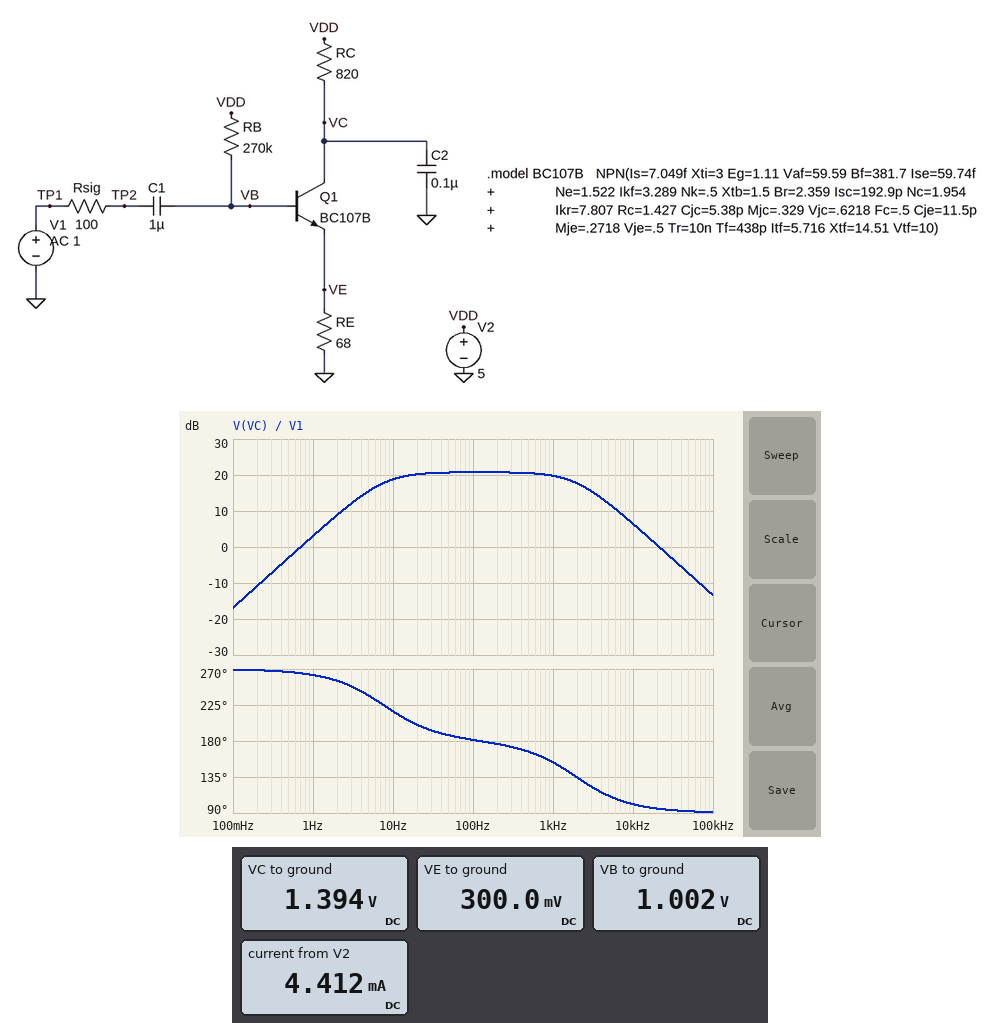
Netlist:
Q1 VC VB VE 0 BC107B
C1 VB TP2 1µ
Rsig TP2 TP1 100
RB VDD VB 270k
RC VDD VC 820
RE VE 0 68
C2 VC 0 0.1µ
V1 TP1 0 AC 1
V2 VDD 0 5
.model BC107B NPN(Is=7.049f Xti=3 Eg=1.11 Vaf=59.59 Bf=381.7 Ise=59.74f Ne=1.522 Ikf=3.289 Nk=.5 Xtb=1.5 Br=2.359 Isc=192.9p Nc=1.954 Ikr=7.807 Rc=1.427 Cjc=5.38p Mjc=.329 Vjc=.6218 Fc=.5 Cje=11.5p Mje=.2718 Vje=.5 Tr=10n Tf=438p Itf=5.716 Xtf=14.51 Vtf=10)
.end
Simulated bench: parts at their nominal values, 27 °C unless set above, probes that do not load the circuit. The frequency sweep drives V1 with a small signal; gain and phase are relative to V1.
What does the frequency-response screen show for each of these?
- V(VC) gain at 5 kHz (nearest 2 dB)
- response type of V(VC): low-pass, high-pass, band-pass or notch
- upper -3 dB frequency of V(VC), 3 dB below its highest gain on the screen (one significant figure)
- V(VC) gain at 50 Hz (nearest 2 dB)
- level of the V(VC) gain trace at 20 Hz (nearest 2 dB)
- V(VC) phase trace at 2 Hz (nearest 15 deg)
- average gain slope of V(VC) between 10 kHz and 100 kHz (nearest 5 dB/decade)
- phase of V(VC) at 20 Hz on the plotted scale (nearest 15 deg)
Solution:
12 dB
band-pass
2 kHz
20 dB
20 dB
255 deg
-20 dB/decade
195 deg
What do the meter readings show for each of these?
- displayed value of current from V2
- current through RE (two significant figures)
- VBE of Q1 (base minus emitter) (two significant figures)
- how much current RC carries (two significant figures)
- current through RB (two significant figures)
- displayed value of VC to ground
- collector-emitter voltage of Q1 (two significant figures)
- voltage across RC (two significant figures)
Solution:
4.412 mA
4.4 mA
700 mV
4.4 mA
15 µA
1.394 V
1.1 V
3.6 V
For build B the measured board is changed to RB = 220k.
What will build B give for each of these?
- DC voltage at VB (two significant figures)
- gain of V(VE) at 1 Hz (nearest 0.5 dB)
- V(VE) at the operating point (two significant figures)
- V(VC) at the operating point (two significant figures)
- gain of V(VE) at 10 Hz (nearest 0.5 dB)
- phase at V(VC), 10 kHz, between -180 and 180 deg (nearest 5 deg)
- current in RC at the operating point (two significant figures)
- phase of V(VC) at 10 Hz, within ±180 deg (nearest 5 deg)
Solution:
1.1 V
-26.0 dB
360 mV
710 mV
-7.0 dB
100 deg
5.2 mA
-120 deg
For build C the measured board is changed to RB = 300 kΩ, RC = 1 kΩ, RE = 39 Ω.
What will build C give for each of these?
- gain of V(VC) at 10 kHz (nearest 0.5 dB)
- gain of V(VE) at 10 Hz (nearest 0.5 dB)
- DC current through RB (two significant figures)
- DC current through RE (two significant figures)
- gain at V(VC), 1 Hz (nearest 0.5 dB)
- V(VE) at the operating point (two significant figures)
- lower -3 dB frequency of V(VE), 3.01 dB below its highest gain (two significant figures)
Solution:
10.5 dB
-5.5 dB
14 µA
4.1 mA
5.0 dB
160 mV
12 Hz
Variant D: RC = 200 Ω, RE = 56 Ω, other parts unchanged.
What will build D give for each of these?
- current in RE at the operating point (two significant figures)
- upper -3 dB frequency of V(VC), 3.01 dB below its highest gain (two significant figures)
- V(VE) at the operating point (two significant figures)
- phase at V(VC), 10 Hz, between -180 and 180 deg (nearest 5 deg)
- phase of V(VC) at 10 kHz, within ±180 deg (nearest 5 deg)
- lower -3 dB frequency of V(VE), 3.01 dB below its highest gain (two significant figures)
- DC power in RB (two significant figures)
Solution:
4.7 mA
8.0 kHz
260 mV
-140 deg
130 deg
8.4 Hz
60 µW
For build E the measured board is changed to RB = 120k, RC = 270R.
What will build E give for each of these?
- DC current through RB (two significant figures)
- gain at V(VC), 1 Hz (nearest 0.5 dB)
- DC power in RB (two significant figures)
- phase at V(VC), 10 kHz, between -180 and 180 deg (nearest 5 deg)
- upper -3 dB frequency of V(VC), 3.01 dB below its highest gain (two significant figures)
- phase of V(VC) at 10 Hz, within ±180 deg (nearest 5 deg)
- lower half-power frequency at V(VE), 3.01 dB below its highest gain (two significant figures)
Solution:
30 µA
-7.0 dB
110 µW
120 deg
5.9 kHz
-140 deg
8.3 Hz
